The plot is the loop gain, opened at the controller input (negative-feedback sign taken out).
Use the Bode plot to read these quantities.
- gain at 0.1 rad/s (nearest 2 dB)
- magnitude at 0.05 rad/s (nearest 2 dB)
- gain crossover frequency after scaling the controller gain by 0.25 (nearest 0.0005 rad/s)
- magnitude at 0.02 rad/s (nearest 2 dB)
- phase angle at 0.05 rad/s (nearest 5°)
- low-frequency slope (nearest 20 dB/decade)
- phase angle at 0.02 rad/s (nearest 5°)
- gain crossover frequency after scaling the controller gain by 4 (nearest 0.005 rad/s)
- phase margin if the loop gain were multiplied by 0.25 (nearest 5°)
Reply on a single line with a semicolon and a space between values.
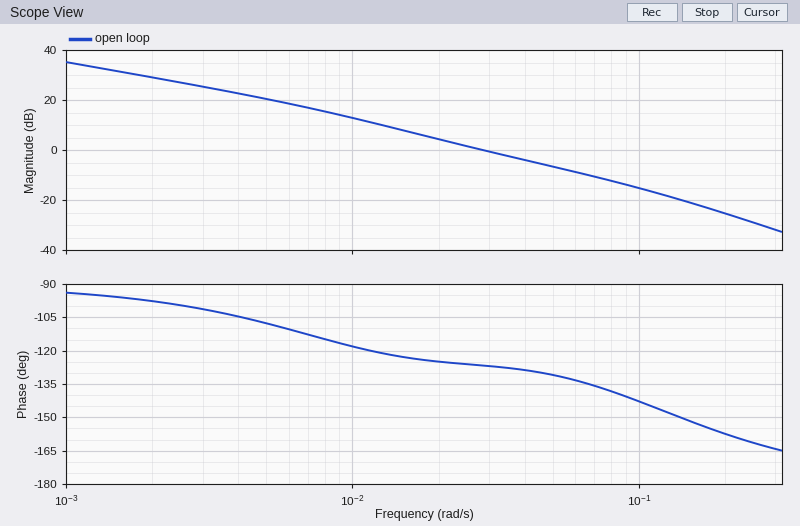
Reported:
-16 dB; -6 dB; 0.0105 rad/s; 4 dB; -130°; -20 dB/decade; -125°; 0.080 rad/s; 60°
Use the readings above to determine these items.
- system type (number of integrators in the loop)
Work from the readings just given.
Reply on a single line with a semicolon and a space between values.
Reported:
1
